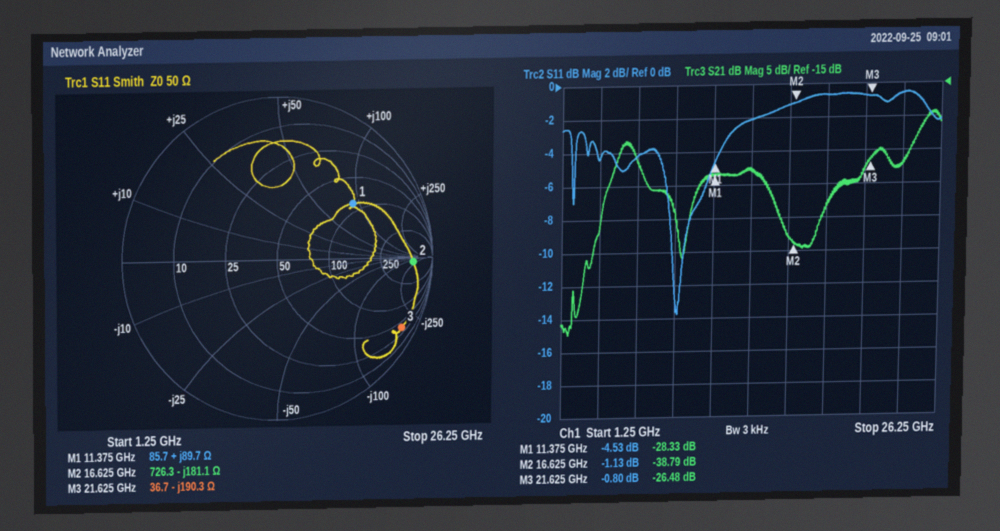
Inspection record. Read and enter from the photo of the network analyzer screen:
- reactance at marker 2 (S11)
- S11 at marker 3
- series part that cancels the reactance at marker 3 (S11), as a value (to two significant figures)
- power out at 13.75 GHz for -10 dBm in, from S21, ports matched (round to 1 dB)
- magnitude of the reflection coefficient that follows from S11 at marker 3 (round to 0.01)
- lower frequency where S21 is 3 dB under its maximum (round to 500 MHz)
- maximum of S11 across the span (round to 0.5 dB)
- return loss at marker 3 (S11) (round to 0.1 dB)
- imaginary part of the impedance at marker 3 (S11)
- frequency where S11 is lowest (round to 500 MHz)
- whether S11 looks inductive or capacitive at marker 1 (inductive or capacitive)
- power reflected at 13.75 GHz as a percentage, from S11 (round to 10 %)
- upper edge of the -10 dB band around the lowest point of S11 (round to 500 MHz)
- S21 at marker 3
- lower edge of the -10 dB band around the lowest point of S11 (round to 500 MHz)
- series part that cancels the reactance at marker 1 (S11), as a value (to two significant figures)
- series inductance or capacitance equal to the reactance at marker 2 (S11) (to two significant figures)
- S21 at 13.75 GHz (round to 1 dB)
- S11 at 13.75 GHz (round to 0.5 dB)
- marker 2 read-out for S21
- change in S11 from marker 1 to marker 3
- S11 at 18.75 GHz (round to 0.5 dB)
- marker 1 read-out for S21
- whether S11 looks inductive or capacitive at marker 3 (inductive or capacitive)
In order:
-181.1 Ω
-0.80 dB
1.4 nH
-38 dBm
0.91
25.0 GHz
-0.5 dB
0.8 dB
-190.3 Ω
9.0 GHz
inductive
60 %
9.5 GHz
-26.48 dB
8.5 GHz
160 fF
53 fF
-28 dB
-2.0 dB
-38.79 dB
3.73 dB
-0.5 dB
-28.33 dB
capacitive
